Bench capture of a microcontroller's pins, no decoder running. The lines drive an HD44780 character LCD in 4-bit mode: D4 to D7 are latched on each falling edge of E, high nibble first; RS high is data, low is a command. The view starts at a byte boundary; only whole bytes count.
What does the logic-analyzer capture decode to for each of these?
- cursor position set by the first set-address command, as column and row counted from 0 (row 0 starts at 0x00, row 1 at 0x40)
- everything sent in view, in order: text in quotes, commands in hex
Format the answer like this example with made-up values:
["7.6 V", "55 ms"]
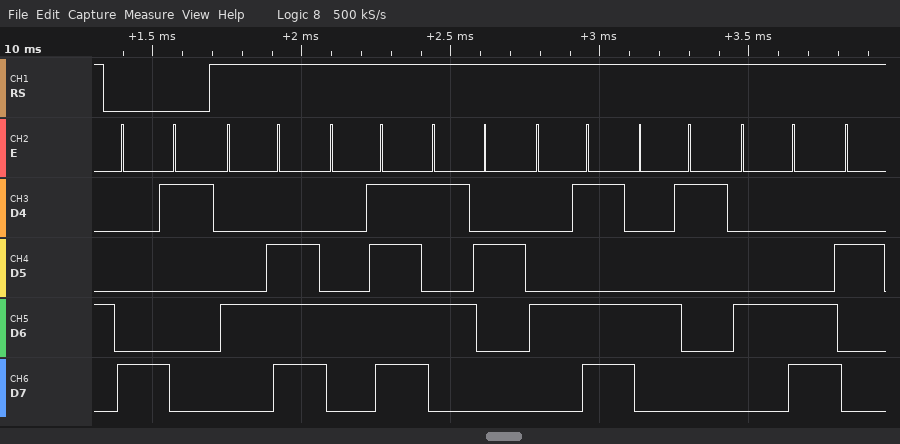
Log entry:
["column 1, row 0", "0x81 \"NORMAL\""]
